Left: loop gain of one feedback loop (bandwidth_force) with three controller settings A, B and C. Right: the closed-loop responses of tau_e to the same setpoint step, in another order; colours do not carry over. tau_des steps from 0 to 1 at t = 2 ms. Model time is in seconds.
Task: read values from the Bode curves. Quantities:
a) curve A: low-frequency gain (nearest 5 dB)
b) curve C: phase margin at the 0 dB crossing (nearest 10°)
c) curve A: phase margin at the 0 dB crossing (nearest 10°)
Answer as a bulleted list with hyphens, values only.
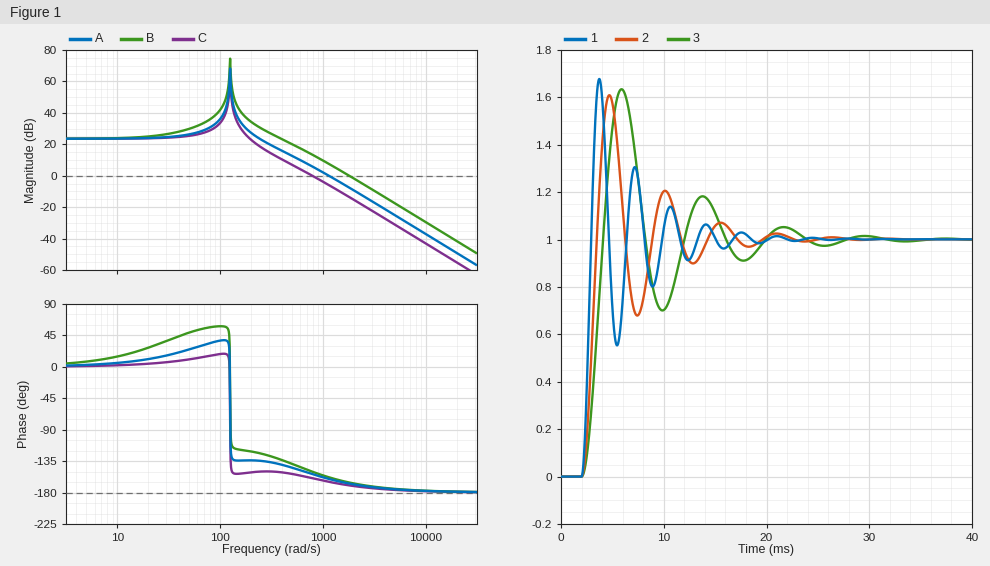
- 25 dB
- 20°
- 20°
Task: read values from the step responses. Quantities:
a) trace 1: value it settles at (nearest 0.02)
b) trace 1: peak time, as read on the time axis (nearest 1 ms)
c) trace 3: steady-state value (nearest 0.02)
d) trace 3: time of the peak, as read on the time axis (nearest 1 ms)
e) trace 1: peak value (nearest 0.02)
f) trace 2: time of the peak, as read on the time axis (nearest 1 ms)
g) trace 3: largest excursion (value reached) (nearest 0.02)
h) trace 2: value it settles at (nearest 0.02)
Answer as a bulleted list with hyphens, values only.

- 1.00
- 4 ms
- 1.00
- 6 ms
- 1.68
- 5 ms
- 1.64
- 1.00
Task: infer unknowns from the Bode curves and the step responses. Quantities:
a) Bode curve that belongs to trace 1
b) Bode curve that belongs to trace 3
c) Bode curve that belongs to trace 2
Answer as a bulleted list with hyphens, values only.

- B
- C
- A
